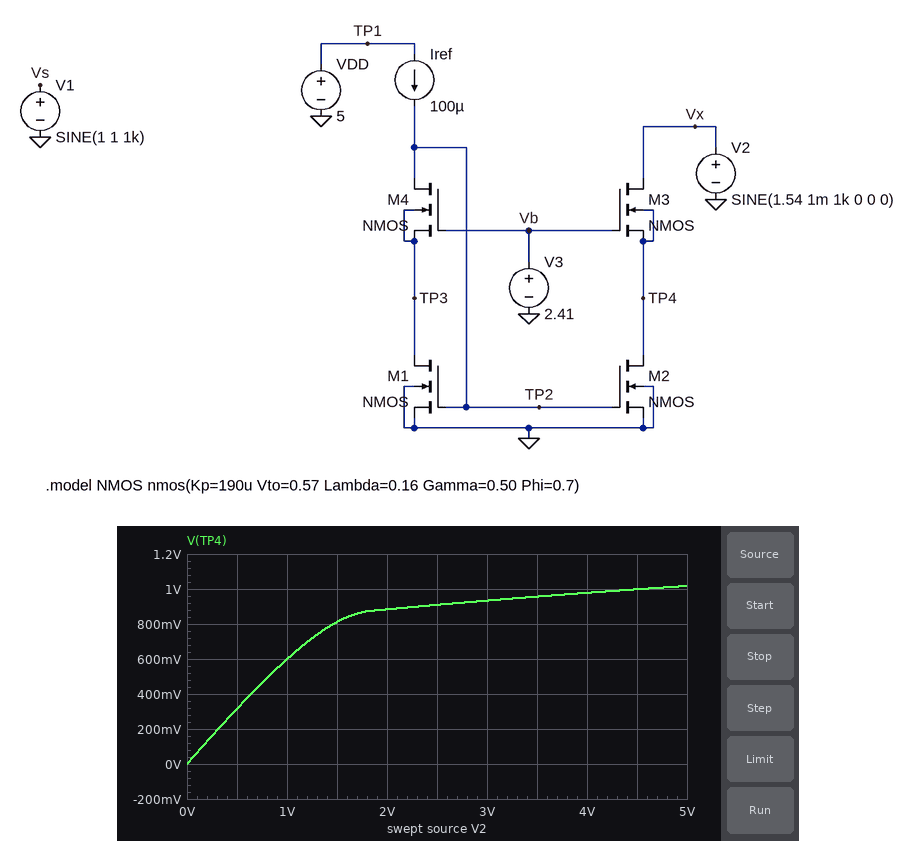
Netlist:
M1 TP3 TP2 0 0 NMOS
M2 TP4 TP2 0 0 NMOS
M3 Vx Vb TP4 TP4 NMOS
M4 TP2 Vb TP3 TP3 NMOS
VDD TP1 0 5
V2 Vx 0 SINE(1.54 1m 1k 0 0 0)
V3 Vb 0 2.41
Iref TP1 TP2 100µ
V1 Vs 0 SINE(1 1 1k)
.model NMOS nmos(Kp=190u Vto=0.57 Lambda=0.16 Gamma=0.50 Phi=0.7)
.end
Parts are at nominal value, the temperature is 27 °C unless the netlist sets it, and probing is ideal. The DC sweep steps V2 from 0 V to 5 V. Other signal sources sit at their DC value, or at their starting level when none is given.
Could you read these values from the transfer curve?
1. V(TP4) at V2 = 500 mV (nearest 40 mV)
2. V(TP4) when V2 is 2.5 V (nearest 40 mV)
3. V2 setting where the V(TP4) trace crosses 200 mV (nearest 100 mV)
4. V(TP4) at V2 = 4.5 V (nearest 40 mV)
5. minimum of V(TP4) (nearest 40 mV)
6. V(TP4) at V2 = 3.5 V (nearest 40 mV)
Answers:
320 mV
920 mV
300 mV
1.00 V
0 V
960 mV
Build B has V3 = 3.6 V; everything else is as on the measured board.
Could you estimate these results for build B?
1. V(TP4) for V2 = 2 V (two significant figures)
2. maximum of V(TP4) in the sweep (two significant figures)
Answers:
1.6 V
2.1 V
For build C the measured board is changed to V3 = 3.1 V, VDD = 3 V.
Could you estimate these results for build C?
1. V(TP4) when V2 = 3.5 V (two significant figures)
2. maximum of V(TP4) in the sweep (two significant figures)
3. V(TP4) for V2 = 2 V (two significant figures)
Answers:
1.6 V
1.7 V
1.4 V
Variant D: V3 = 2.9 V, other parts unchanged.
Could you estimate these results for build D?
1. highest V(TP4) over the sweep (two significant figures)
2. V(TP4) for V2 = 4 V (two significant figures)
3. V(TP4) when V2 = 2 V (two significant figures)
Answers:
1.5 V
1.4 V
1.3 V
